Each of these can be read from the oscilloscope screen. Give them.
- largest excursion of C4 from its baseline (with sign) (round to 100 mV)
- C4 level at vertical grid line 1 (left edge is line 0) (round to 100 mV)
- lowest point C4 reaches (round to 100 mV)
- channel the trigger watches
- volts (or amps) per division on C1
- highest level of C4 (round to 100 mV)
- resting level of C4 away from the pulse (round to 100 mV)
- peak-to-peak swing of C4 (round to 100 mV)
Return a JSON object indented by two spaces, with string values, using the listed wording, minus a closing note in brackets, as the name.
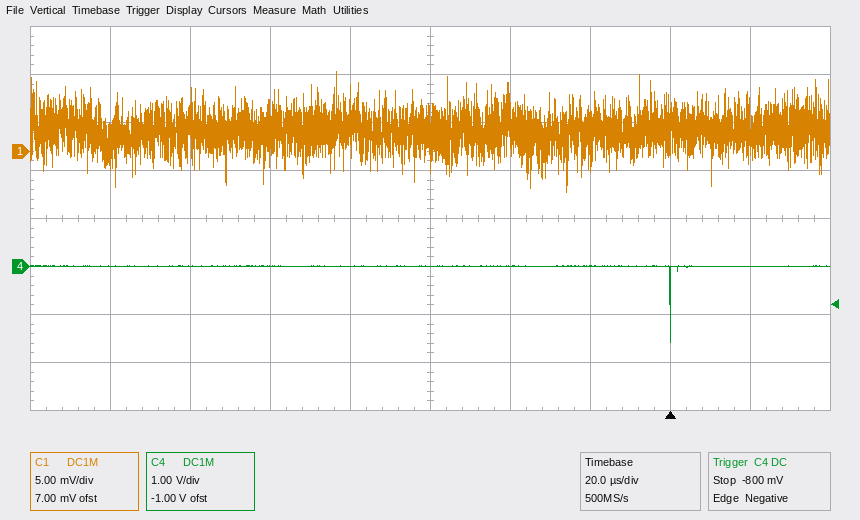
{
  "largest excursion of C4 from its baseline (with sign)": "-1.6 V",
  "C4 level at vertical grid line 1 (left edge is line 0)": "0.0 V",
  "lowest point C4 reaches": "-1.6 V",
  "channel the trigger watches": "C4",
  "volts (or amps) per division on C1": "5 mV",
  "highest level of C4": "0.0 V",
  "resting level of C4 away from the pulse": "0.0 V",
  "peak-to-peak swing of C4": "1.6 V"
}
